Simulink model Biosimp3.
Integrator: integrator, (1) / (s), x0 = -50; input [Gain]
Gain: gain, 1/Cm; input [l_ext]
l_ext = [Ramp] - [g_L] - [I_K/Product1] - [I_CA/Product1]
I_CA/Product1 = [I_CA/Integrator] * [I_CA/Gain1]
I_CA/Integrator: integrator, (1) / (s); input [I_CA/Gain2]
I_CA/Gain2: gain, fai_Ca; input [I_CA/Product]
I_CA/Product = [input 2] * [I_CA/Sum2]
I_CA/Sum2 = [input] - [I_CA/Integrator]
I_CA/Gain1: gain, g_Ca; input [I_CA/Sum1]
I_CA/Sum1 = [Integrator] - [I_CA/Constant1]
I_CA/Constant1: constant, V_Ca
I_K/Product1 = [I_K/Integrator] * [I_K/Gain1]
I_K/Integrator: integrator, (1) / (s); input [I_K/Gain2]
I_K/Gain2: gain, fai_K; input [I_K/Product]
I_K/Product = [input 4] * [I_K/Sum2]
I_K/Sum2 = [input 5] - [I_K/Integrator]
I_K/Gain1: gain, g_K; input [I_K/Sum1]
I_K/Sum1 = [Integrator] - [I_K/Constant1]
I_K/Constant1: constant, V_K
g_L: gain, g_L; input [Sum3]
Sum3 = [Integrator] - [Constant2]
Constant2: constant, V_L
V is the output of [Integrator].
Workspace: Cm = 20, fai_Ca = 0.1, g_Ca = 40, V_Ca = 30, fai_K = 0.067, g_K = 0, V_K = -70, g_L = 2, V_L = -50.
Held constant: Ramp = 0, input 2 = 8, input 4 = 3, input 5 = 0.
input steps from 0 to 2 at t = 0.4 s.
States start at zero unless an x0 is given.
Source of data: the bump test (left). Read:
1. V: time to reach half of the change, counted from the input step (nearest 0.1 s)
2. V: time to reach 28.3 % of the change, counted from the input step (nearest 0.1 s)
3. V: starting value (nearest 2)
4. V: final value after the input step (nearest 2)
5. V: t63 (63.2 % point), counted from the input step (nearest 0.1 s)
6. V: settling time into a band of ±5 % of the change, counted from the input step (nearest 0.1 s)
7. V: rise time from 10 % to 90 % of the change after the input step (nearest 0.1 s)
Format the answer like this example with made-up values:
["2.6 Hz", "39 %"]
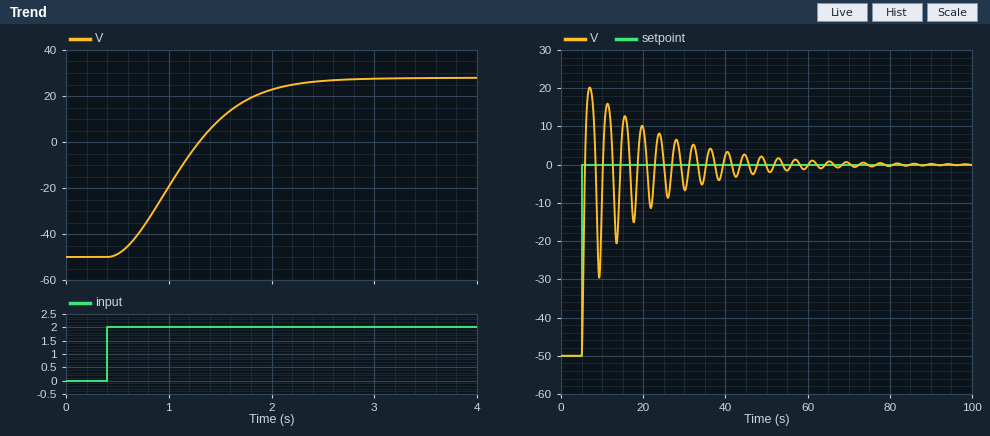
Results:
["0.7 s", "0.5 s", "-50", "28", "0.9 s", "1.7 s", "1.2 s"]
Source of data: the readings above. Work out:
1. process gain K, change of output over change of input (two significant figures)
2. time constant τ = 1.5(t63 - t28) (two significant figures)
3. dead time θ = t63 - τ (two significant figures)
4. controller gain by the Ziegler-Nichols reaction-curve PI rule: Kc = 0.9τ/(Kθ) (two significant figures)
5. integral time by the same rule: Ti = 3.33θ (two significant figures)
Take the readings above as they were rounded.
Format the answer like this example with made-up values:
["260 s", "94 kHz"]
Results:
["39", "0.60 s", "0.30 s", "0.046", "1.00 s"]
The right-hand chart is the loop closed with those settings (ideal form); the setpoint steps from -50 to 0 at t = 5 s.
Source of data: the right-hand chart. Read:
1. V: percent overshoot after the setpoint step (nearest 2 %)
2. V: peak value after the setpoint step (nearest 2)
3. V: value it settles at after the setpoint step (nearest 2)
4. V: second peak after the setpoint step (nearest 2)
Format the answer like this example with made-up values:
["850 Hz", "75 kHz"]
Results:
["40 %", "20", "0", "16"]
